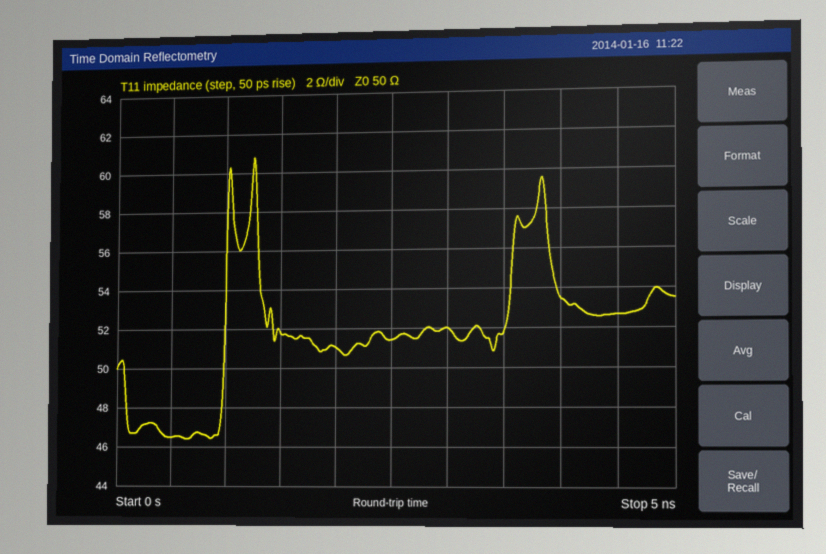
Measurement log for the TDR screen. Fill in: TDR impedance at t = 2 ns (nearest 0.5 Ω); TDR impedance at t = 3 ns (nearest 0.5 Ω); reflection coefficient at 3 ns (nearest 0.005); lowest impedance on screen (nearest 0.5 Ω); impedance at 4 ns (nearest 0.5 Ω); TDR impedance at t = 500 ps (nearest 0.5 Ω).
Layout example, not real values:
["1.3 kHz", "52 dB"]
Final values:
["51.0 Ω", "52.0 Ω", "+0.020", "46.5 Ω", "53.5 Ω", "46.5 Ω"]
